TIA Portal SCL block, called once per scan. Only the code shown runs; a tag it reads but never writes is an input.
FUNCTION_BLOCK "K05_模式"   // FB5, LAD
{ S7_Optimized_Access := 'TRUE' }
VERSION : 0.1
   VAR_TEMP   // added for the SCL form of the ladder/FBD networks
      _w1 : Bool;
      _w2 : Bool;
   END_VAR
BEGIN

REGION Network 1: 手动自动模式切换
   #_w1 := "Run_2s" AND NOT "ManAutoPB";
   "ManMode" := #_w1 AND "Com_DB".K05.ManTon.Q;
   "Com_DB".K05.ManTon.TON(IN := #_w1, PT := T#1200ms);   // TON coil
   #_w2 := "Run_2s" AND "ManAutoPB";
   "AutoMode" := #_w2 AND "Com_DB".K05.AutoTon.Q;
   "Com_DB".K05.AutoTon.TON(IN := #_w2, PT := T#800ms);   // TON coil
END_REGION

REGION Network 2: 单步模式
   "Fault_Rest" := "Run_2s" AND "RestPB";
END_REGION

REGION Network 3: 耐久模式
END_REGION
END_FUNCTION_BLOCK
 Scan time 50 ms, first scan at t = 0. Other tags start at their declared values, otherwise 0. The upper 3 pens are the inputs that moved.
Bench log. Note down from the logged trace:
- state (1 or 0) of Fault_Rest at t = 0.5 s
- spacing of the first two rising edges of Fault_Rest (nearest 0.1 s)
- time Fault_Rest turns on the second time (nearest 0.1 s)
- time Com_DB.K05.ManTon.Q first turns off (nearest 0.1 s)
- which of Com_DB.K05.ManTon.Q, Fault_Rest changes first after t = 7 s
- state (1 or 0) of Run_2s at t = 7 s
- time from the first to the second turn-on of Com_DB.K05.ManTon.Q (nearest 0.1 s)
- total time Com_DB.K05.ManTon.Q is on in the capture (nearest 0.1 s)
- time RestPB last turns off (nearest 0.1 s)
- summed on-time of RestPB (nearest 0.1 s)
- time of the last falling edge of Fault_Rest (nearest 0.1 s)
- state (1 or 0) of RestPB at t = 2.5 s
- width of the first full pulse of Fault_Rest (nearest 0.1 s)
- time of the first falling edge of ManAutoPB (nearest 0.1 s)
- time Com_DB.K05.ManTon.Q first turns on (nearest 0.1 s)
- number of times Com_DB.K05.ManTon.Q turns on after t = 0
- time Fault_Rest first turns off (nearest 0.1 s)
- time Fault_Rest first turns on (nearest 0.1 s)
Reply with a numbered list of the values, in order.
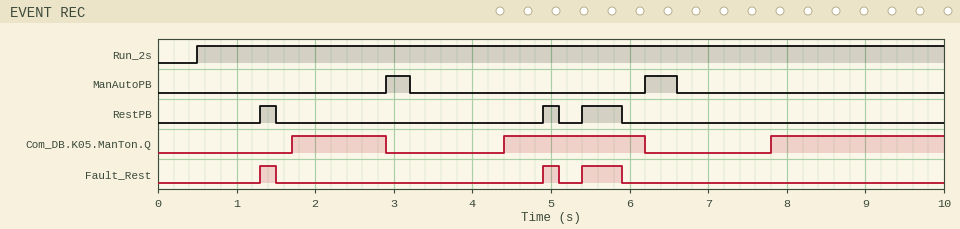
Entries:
1. 0
2. 3.6 s
3. 4.9 s
4. 2.9 s
5. Com_DB.K05.ManTon.Q
6. 1
7. 2.7 s
8. 5.2 s
9. 5.9 s
10. 0.9 s
11. 5.9 s
12. 0
13. 0.2 s
14. 3.2 s
15. 1.7 s
16. 3
17. 1.5 s
18. 1.3 s
